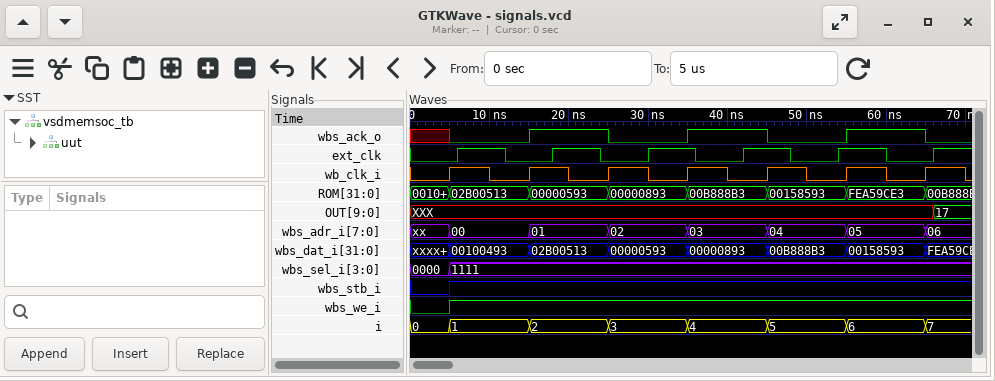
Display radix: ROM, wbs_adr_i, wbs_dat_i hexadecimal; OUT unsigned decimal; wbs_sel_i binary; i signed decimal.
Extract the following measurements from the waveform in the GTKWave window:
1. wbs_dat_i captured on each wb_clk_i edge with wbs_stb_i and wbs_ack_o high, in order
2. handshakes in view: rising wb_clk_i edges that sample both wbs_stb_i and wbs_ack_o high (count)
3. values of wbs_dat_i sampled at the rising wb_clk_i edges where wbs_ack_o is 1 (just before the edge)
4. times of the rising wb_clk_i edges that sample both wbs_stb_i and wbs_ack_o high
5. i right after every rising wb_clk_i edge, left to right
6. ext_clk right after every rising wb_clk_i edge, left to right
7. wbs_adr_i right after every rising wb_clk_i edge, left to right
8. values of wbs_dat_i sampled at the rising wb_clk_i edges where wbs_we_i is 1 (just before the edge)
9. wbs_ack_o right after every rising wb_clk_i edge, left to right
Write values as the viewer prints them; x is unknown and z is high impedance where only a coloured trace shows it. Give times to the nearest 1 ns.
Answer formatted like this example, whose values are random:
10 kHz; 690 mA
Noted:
02B00513, 00000893, 00158593; 3; 02B00513, 00000893, 00158593; 25 ns, 45 ns, 65 ns; 1, 2, 3, 4, 5, 6, 7; 0 0 0 1 1 1 0; 00, 01, 02, 03, 04, 05, 06; 00100493, 02B00513, 00000593, 00000893, 00B888B3, 00158593; 0 1 0 1 0 1 0
